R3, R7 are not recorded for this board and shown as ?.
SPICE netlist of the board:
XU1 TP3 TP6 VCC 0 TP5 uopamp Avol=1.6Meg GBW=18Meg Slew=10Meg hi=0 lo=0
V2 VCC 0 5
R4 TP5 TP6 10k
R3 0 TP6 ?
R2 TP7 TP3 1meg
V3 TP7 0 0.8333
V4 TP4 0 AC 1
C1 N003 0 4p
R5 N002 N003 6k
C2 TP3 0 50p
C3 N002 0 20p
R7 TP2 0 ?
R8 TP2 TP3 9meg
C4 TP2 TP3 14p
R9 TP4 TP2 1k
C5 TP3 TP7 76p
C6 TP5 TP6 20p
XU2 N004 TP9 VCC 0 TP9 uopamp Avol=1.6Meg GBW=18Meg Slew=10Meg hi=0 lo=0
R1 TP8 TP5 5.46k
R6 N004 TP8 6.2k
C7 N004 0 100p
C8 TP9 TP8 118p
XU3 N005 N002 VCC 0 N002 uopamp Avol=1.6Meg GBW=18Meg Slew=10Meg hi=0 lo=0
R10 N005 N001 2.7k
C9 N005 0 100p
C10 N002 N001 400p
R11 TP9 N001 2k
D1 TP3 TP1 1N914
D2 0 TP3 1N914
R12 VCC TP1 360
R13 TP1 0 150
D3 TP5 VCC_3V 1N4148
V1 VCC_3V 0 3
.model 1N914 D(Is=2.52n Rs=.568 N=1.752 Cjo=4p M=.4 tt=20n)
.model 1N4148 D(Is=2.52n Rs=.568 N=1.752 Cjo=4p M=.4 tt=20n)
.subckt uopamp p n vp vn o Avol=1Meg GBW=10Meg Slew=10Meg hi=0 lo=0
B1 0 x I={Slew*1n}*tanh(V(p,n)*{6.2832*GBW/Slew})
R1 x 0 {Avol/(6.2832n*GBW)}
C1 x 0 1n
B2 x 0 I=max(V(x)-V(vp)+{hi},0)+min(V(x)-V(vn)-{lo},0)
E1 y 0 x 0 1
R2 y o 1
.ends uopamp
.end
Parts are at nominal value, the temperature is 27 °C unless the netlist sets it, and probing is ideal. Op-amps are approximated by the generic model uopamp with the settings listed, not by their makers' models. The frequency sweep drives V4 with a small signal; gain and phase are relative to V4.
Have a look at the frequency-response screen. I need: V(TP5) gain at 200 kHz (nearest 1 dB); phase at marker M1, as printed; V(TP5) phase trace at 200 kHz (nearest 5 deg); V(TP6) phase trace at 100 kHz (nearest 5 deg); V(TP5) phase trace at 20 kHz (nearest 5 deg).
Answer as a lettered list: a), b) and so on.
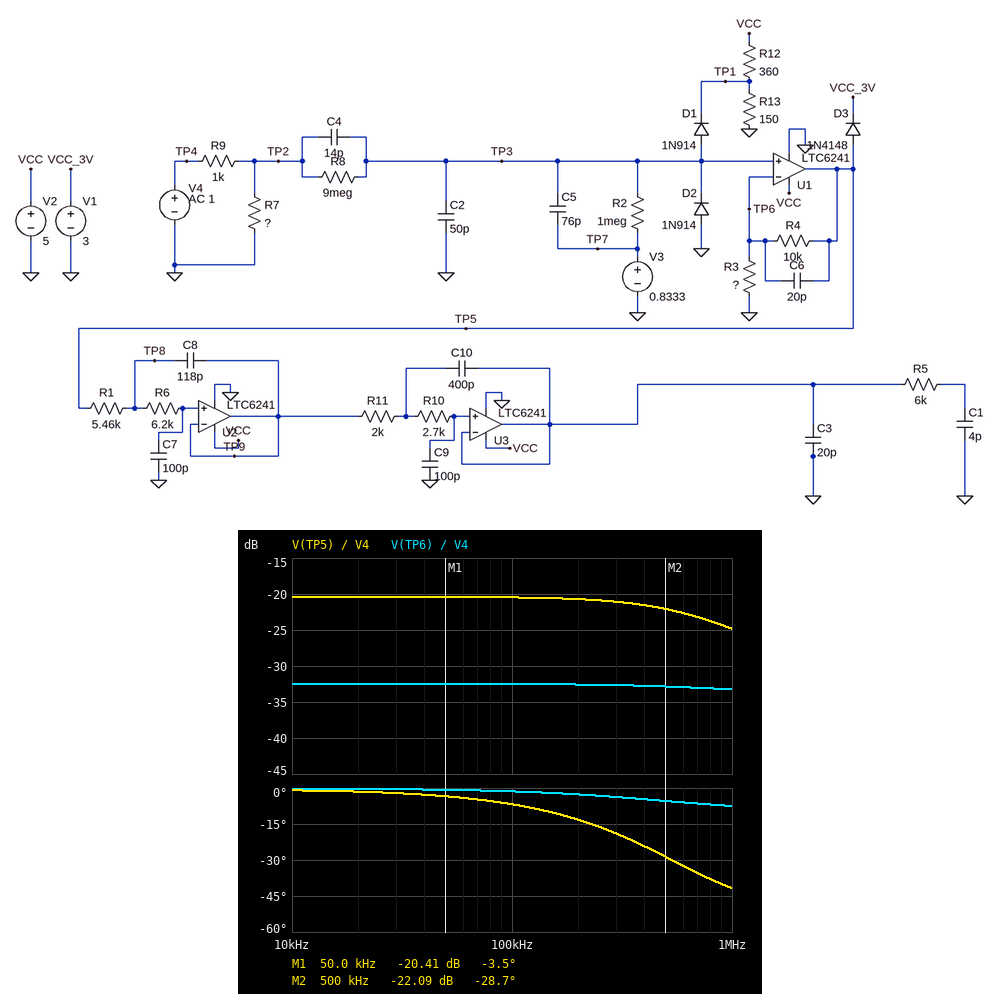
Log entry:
a) -21 dB
b) -3.5 deg
c) -15 deg
d) 0 deg
e) 0 deg
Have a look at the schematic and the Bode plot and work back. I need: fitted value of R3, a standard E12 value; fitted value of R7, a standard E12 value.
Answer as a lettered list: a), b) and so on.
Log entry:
a) 3.3 kΩ
b) 330 Ω
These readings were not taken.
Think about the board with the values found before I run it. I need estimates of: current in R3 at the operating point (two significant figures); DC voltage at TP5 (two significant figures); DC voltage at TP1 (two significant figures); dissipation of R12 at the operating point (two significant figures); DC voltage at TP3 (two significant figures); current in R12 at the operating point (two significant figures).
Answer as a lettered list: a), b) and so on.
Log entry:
a) 230 µA
b) 3.0 V
c) 1.5 V
d) 35 mW
e) 750 mV
f) 9.8 mA
